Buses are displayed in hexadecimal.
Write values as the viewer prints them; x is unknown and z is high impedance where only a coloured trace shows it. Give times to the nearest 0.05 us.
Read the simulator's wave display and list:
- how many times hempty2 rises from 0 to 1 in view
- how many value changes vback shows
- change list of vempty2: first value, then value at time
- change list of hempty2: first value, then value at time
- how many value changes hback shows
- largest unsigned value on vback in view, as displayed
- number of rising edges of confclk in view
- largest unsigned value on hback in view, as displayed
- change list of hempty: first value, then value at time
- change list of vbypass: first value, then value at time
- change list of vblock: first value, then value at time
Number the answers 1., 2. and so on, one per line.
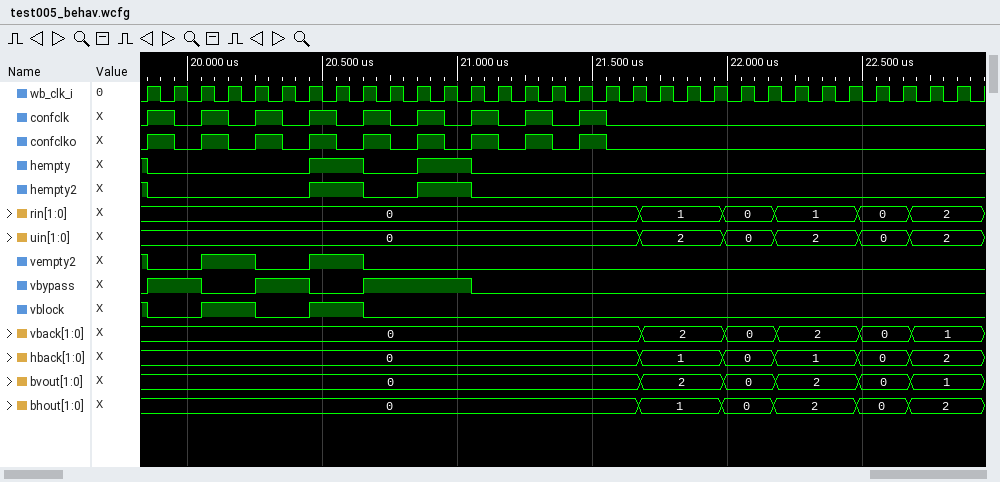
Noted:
1. 2
2. 5
3. 1, 0 at 19.85 us, 1 at 20.05 us, 0 at 20.25 us, 1 at 20.45 us, 0 at 20.65 us
4. 1, 0 at 19.85 us, 1 at 20.45 us, 0 at 20.65 us, 1 at 20.85 us, 0 at 21.05 us
5. 5
6. 2
7. 9
8. 2
9. 1, 0 at 19.85 us, 1 at 20.45 us, 0 at 20.65 us, 1 at 20.85 us, 0 at 21.05 us
10. 0, 1 at 19.85 us, 0 at 20.05 us, 1 at 20.25 us, 0 at 20.45 us, 1 at 20.65 us, 0 at 21.05 us
11. 1, 0 at 19.85 us, 1 at 20.05 us, 0 at 20.25 us, 1 at 20.45 us, 0 at 20.65 us
